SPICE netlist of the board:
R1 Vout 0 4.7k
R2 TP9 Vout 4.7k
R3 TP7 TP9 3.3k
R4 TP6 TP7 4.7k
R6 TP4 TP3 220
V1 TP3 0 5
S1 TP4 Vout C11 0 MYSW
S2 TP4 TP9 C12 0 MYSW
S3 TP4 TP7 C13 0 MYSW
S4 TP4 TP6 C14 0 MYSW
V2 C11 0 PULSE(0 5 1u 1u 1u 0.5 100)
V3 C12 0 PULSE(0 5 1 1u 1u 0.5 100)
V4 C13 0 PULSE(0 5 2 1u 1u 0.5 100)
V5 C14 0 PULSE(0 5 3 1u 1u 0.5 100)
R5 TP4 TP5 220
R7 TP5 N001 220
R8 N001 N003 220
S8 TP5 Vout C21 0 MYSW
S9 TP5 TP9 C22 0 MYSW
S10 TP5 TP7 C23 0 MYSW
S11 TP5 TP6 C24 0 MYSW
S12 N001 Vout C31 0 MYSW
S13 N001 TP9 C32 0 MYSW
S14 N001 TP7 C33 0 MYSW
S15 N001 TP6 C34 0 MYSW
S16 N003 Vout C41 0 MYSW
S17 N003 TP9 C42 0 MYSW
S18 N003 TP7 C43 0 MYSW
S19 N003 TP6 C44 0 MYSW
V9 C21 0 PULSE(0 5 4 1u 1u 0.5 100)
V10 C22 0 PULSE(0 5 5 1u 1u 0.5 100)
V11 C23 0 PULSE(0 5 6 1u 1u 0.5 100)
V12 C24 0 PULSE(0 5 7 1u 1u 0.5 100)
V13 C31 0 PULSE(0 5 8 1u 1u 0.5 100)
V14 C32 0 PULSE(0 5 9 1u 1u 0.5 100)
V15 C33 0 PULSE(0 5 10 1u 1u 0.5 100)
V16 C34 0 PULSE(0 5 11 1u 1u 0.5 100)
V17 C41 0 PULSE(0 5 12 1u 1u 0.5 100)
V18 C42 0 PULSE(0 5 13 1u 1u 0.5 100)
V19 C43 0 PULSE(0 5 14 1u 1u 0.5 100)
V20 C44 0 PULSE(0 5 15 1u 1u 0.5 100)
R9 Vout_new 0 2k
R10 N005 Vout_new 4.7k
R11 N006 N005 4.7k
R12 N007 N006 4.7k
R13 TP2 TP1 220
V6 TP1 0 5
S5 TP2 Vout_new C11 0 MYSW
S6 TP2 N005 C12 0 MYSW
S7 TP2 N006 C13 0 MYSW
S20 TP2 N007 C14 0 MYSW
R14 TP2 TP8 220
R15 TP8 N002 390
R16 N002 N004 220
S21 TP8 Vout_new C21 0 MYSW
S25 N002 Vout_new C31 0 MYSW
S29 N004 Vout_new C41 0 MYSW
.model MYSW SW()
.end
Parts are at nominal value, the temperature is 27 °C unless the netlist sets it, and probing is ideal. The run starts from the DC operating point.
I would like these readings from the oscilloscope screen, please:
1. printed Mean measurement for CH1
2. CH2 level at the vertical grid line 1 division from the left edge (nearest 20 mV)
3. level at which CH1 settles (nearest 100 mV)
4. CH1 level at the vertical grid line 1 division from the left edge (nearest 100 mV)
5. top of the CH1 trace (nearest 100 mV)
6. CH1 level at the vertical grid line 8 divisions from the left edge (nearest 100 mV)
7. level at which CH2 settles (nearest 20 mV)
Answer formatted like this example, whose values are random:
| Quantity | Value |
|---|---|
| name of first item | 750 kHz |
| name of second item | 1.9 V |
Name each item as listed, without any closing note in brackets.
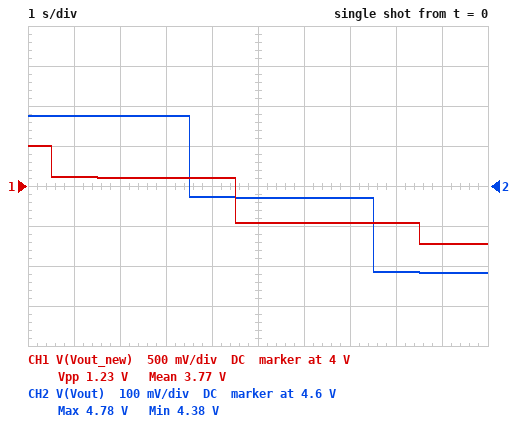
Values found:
| Quantity | Value |
|---|---|
| printed Mean measurement for CH1 | 3.77 V |
| CH2 level at the vertical grid line 1 division from the left edge | 4.78 V |
| level at which CH1 settles | 3.3 V |
| CH1 level at the vertical grid line 1 division from the left edge | 4.1 V |
| top of the CH1 trace | 4.5 V |
| CH1 level at the vertical grid line 8 divisions from the left edge | 3.5 V |
| level at which CH2 settles | 4.38 V |
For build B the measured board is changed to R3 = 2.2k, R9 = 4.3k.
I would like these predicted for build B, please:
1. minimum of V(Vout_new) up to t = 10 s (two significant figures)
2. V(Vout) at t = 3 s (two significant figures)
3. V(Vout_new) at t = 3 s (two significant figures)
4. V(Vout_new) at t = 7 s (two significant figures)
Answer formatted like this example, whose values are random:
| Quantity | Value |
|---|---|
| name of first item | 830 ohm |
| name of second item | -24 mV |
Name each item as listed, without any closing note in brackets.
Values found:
| Quantity | Value |
|---|---|
| minimum of V(Vout_new) up to t = 10 s | 4.0 V |
| V(Vout) at t = 3 s | 4.8 V |
| V(Vout_new) at t = 3 s | 4.5 V |
| V(Vout_new) at t = 7 s | 4.2 V |
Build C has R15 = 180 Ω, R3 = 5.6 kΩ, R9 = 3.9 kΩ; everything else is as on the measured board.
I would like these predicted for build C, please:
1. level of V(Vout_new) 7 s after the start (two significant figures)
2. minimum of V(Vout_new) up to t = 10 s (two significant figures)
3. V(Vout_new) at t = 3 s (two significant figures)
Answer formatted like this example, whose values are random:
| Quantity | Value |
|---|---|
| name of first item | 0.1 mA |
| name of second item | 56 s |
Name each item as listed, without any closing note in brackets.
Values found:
| Quantity | Value |
|---|---|
| level of V(Vout_new) 7 s after the start | 4.3 V |
| minimum of V(Vout_new) up to t = 10 s | 4.1 V |
| V(Vout_new) at t = 3 s | 4.5 V |
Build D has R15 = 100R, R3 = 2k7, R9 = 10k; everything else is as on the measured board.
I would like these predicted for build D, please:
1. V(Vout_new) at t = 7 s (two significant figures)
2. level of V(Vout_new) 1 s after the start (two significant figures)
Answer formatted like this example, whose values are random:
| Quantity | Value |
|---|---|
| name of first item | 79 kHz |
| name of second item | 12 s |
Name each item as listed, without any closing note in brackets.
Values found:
| Quantity | Value |
|---|---|
| V(Vout_new) at t = 7 s | 4.7 V |
| level of V(Vout_new) 1 s after the start | 4.8 V |
